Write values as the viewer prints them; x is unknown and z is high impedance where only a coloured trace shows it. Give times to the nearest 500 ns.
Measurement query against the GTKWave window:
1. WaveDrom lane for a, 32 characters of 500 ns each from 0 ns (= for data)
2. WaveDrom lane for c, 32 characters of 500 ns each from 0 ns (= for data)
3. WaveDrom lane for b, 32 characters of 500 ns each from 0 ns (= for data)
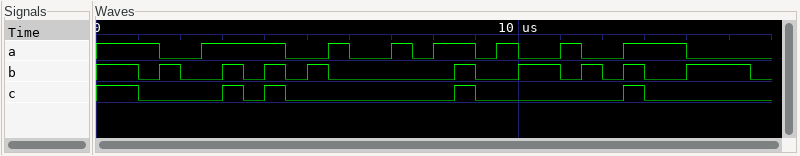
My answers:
{name: 'a', wave: '1..0.1...0.10.101.010.10.1..0...'}
{name: 'c', wave: '1.0...1010.......10......10.....'}
{name: 'b', wave: '1.010.101010.....10.1.01010.1..0'}
